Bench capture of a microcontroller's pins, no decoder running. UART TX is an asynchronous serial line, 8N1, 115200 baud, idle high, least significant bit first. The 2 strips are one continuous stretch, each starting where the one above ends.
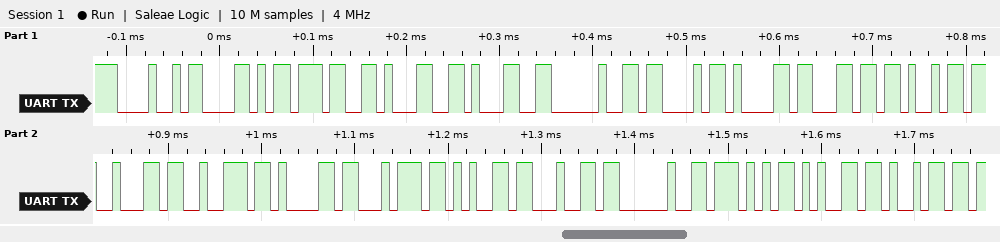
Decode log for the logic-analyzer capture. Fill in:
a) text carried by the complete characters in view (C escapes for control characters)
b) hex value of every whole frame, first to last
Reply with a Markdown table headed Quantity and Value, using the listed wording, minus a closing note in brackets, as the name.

| Quantity | Value |
|---|---|
| text carried by the complete characters in view | "HX711 Calibrated Wei" |
| hex value of every whole frame, first to last | 48 58 37 31 31 20 43 61 6C 69 62 72 61 74 65 64 20 57 65 69 |
